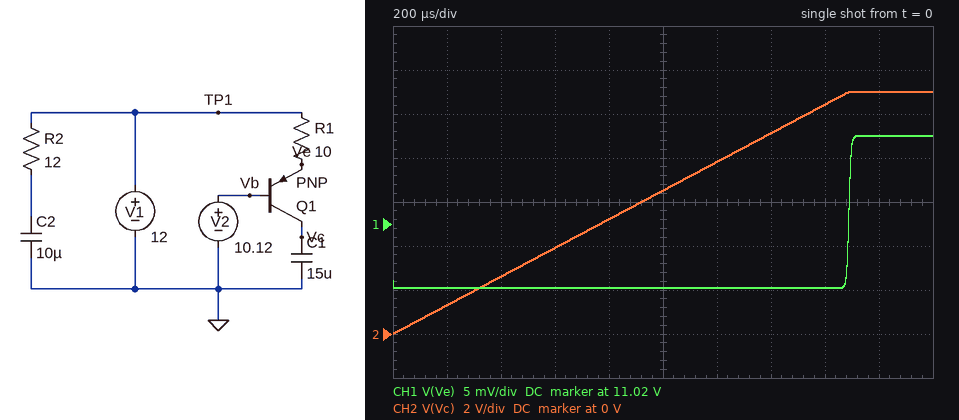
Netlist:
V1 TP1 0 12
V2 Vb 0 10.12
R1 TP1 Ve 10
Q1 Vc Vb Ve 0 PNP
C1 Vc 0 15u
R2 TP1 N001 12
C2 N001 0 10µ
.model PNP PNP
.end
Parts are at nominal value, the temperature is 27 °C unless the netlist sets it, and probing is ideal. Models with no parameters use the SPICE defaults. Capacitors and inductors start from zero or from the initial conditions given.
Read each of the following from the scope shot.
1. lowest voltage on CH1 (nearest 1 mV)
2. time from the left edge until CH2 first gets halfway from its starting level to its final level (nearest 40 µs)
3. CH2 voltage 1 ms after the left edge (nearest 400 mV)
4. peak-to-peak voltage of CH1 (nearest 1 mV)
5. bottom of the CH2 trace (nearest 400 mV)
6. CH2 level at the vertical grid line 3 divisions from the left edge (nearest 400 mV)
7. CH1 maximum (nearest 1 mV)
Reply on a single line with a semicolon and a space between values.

11.013 V; 840 µs; 6.4 V; 17 mV; 0 V; 4.0 V; 11.030 V
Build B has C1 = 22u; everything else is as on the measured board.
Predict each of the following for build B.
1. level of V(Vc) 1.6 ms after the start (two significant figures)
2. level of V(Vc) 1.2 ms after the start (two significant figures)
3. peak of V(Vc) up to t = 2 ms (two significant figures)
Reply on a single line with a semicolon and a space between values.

7.1 V; 5.3 V; 8.9 V
